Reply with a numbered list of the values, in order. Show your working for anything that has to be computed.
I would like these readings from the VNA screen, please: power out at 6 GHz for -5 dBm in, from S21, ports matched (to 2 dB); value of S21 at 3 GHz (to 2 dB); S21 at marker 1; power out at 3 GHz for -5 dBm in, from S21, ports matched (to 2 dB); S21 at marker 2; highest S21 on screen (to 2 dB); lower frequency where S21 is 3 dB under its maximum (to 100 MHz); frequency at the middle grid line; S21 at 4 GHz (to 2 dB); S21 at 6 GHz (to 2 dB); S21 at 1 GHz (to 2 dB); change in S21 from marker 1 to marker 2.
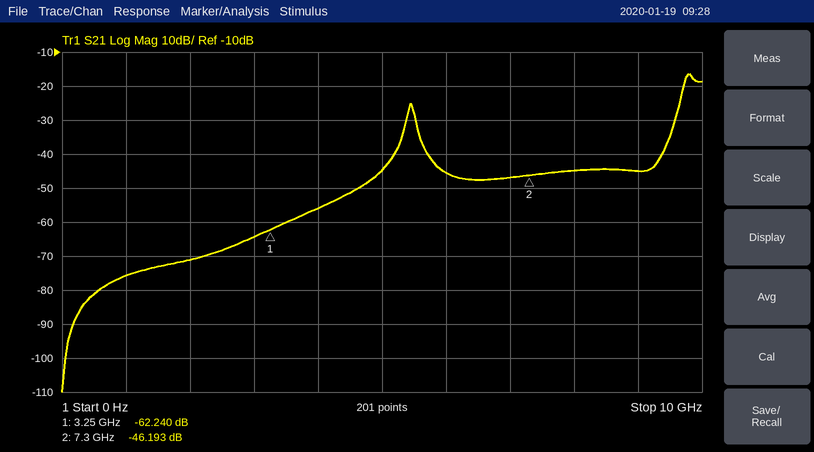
1. -5 dBm + (-46 dB) = -50 dBm
2. -64 dB
3. -62.240 dB
4. -5 dBm + (-64 dB) = -70 dBm
5. -46.193 dB
6. -16 dB
7. 9.7 GHz
8. 5 GHz
9. -56 dB
10. -46 dB
11. -76 dB
12. -46.193 − (-62.24) = 16.047 dB
